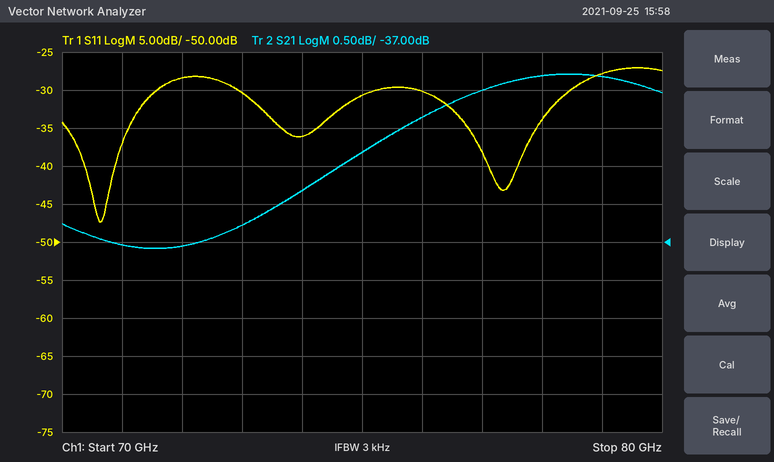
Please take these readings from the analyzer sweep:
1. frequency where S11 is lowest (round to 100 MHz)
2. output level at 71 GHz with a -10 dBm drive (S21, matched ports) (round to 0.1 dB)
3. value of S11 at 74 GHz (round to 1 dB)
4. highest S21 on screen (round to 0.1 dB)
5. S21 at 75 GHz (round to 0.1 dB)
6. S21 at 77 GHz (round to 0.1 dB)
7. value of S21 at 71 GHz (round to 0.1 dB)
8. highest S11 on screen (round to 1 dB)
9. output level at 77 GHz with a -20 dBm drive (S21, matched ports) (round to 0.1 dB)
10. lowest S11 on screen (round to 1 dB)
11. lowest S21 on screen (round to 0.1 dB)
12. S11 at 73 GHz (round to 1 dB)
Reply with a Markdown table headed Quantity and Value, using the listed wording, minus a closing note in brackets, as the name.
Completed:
| Quantity | Value |
|---|---|
| frequency where S11 is lowest | 70.6 GHz |
| output level at 71 GHz with a -10 dBm drive (S21, matched ports) | -47.0 dBm |
| value of S11 at 74 GHz | -36 dB |
| highest S21 on screen | -34.8 dB |
| S21 at 75 GHz | -35.8 dB |
| S21 at 77 GHz | -35.0 dB |
| value of S21 at 71 GHz | -37.0 dB |
| highest S11 on screen | -27 dB |
| output level at 77 GHz with a -20 dBm drive (S21, matched ports) | -55.0 dBm |
| lowest S11 on screen | -47 dB |
| lowest S21 on screen | -37.1 dB |
| S11 at 73 GHz | -30 dB |
